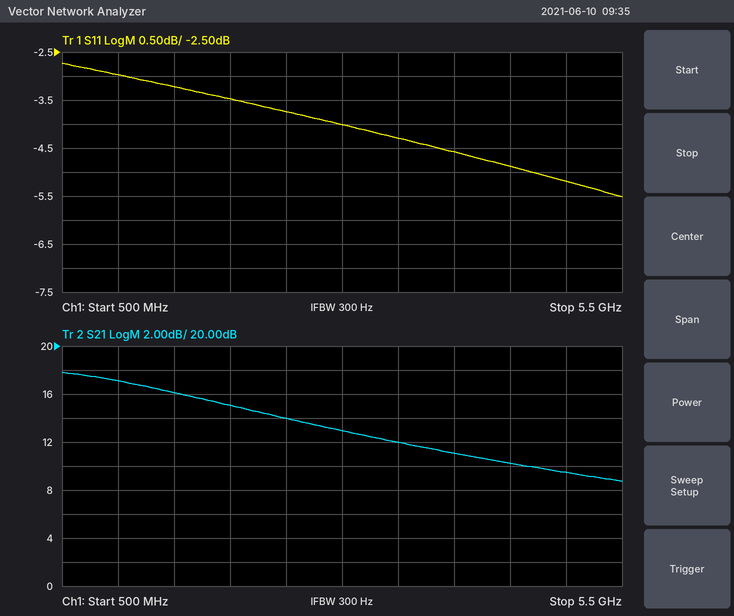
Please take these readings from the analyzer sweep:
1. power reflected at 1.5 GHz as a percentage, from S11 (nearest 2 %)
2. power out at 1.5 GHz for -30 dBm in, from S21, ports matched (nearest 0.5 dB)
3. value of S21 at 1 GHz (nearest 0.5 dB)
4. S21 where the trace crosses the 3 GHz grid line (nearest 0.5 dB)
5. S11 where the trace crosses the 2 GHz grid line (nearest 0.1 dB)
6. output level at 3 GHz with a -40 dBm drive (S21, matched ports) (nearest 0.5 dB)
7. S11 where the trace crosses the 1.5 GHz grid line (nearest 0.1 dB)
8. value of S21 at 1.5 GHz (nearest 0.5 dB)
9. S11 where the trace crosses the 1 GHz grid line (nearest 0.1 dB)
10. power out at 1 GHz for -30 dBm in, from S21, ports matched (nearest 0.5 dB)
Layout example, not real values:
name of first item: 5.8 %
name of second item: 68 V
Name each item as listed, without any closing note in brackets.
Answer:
power reflected at 1.5 GHz as a percentage, from S11: 48 %
power out at 1.5 GHz for -30 dBm in, from S21, ports matched: -14.0 dBm
value of S21 at 1 GHz: 17.0 dB
S21 where the trace crosses the 3 GHz grid line: 13.0 dB
S11 where the trace crosses the 2 GHz grid line: -3.5 dB
output level at 3 GHz with a -40 dBm drive (S21, matched ports): -27.0 dBm
S11 where the trace crosses the 1.5 GHz grid line: -3.2 dB
value of S21 at 1.5 GHz: 16.0 dB
S11 where the trace crosses the 1 GHz grid line: -3.0 dB
power out at 1 GHz for -30 dBm in, from S21, ports matched: -13.0 dBm
